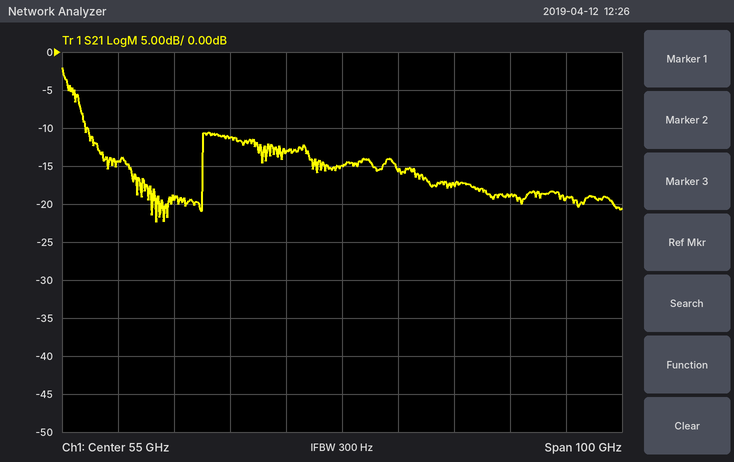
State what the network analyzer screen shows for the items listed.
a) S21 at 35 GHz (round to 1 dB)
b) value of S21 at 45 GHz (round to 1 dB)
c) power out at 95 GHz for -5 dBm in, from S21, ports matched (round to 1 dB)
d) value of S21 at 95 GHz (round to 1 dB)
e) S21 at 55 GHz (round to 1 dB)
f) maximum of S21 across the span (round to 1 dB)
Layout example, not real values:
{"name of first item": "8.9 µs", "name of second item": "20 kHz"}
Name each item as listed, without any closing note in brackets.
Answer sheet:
{"S21 at 35 GHz": "-11 dB", "value of S21 at 45 GHz": "-13 dB", "power out at 95 GHz for -5 dBm in, from S21, ports matched": "-24 dBm", "value of S21 at 95 GHz": "-19 dB", "S21 at 55 GHz": "-15 dB", "maximum of S21 across the span": "-2 dB"}
